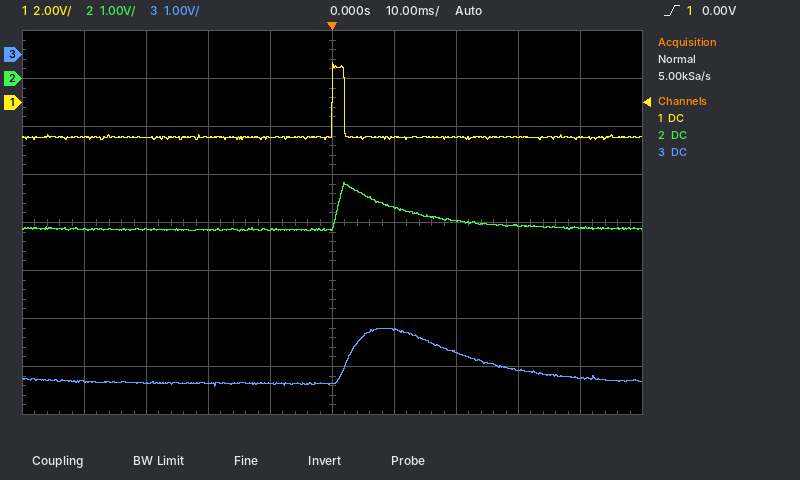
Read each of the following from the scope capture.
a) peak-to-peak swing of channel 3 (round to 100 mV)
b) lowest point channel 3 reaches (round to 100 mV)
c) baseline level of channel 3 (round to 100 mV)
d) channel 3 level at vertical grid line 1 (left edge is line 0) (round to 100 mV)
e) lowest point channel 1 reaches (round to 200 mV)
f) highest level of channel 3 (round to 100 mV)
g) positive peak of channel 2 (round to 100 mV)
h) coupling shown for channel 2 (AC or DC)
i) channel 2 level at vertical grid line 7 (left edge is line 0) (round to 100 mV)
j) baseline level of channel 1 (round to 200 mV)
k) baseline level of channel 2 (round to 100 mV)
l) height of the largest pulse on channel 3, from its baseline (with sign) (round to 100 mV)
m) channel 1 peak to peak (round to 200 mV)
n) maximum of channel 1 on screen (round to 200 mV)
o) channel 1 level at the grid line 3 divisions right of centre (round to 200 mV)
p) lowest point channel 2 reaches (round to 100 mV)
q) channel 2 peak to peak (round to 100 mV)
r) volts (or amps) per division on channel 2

1.2 V
-6.9 V
-6.8 V
-6.8 V
-1.6 V
-5.7 V
-2.2 V
DC
-3.0 V
-1.4 V
-3.1 V
+1.1 V
3.2 V
1.6 V
-1.4 V
-3.2 V
1.0 V
1 V
